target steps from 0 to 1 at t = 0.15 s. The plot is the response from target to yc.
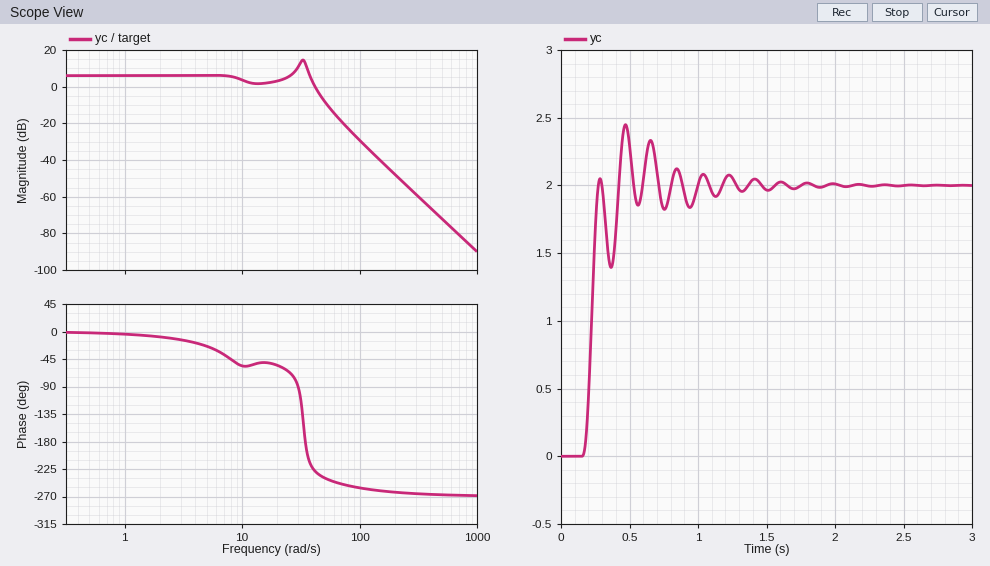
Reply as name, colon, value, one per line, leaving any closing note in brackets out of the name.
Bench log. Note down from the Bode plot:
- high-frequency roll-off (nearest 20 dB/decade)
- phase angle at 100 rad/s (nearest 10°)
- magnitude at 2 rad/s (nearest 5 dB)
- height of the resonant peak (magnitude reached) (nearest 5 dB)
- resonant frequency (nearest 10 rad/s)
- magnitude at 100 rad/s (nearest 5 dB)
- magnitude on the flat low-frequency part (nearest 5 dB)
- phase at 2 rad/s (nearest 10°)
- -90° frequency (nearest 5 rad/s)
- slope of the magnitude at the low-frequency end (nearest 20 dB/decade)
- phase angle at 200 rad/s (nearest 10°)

high-frequency roll-off: -60 dB/decade
phase angle at 100 rad/s: -260°
magnitude at 2 rad/s: 5 dB
height of the resonant peak (magnitude reached): 15 dB
resonant frequency: 30 rad/s
magnitude at 100 rad/s: -30 dB
magnitude on the flat low-frequency part: 5 dB
phase at 2 rad/s: -10°
-90° frequency: 30 rad/s
slope of the magnitude at the low-frequency end: 0 dB/decade
phase angle at 200 rad/s: -260°
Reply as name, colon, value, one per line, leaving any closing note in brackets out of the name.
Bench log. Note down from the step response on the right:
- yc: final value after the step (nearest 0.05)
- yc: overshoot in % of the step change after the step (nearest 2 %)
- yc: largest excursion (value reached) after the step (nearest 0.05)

yc: final value after the step: 2.00
yc: overshoot in % of the step change after the step: 22 %
yc: largest excursion (value reached) after the step: 2.45
